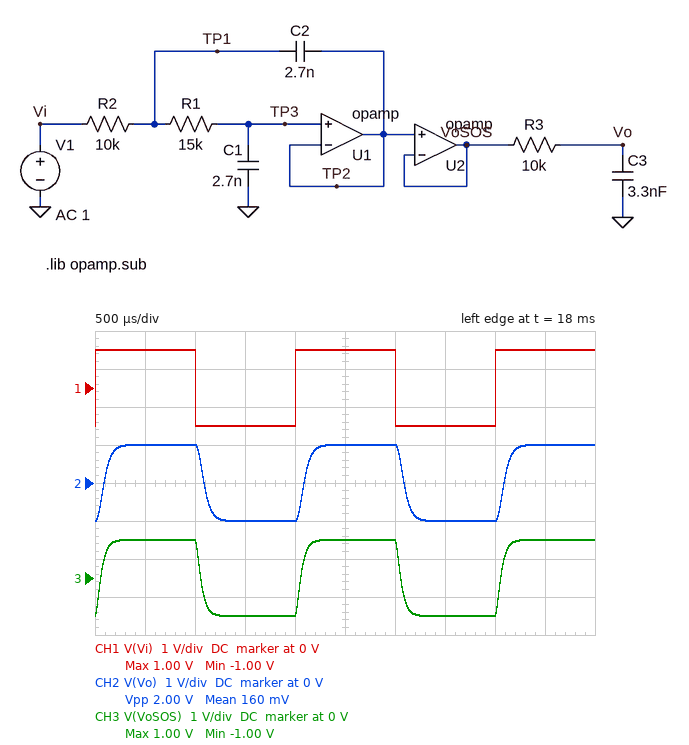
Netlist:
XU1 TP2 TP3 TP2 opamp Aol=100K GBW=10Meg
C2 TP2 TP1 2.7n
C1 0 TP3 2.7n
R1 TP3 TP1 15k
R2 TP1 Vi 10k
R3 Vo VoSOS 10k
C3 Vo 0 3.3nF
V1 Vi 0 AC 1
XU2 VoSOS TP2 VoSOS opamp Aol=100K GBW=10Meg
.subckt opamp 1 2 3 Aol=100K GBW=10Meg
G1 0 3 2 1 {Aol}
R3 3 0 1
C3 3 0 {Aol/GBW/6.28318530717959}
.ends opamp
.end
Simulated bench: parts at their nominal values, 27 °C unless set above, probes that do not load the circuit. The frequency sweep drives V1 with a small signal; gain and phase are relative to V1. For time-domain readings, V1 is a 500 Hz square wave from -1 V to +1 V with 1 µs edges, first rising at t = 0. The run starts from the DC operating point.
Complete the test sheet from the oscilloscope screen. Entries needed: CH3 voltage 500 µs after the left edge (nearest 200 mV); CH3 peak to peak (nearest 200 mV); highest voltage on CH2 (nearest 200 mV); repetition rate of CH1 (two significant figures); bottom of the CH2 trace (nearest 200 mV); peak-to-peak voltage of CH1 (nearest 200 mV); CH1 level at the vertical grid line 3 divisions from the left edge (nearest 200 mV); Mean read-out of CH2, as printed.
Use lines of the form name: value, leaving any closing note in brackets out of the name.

CH3 voltage 500 µs after the left edge: 1.0 V
CH3 peak to peak: 2.0 V
highest voltage on CH2: 1.0 V
repetition rate of CH1: 500 Hz
bottom of the CH2 trace: -1.0 V
peak-to-peak voltage of CH1: 2.0 V
CH1 level at the vertical grid line 3 divisions from the left edge: -1.0 V
Mean read-out of CH2, as printed: 160 mV
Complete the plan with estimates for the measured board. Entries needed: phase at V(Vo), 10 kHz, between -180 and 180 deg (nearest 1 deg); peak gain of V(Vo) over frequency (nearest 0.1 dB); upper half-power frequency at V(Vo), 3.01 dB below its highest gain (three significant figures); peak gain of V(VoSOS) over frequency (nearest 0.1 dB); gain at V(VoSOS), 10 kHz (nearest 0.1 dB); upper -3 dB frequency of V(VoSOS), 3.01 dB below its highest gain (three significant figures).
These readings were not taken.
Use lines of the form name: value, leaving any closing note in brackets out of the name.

phase at V(Vo), 10 kHz, between -180 and 180 deg: 168 deg
peak gain of V(Vo) over frequency: 0 dB
upper half-power frequency at V(Vo), 3.01 dB below its highest gain: 2.40 kHz
peak gain of V(VoSOS) over frequency: 0 dB
gain at V(VoSOS), 10 kHz: -14.6 dB
upper -3 dB frequency of V(VoSOS), 3.01 dB below its highest gain: 3.01 kHz
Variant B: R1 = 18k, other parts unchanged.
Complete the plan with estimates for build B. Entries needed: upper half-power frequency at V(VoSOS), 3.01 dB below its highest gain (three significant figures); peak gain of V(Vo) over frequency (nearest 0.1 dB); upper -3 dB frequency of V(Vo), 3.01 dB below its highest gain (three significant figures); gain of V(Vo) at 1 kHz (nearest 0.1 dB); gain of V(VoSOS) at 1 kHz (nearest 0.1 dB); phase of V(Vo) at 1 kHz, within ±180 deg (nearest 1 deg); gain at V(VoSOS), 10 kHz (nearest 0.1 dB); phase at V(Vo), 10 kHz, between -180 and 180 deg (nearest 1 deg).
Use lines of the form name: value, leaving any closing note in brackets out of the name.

upper half-power frequency at V(VoSOS), 3.01 dB below its highest gain: 2.66 kHz
peak gain of V(Vo) over frequency: 0 dB
upper -3 dB frequency of V(Vo), 3.01 dB below its highest gain: 2.20 kHz
gain of V(Vo) at 1 kHz: -0.7 dB
gain of V(VoSOS) at 1 kHz: -0.5 dB
phase of V(Vo) at 1 kHz, within ±180 deg: -38 deg
gain at V(VoSOS), 10 kHz: -16.0 dB
phase at V(Vo), 10 kHz, between -180 and 180 deg: 164 deg
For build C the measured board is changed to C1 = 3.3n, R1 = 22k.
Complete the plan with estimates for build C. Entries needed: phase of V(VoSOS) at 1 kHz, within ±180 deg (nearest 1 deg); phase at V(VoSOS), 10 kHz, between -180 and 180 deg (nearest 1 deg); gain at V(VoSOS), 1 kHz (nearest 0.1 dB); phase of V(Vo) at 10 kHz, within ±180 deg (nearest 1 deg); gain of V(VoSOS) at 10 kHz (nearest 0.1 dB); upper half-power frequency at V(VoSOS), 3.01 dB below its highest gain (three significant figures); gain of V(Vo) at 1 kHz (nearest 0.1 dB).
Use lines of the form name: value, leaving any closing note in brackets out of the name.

phase of V(VoSOS) at 1 kHz, within ±180 deg: -36 deg
phase at V(VoSOS), 10 kHz, between -180 and 180 deg: -136 deg
gain at V(VoSOS), 1 kHz: -1.1 dB
phase of V(Vo) at 10 kHz, within ±180 deg: 160 deg
gain of V(VoSOS) at 10 kHz: -19.5 dB
upper half-power frequency at V(VoSOS), 3.01 dB below its highest gain: 1.81 kHz
gain of V(Vo) at 1 kHz: -1.3 dB
